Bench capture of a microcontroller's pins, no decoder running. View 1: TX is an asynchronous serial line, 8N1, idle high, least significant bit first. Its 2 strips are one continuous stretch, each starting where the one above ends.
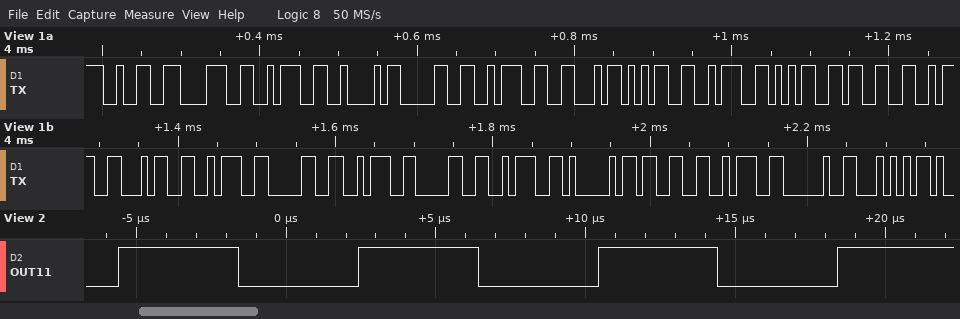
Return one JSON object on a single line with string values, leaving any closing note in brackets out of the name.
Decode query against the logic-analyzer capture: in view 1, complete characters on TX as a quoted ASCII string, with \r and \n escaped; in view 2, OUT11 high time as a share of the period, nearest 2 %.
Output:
{"in view 1, complete characters on TX as a quoted ASCII string, with \\r and \\n escaped": "\"28:B0:F5:53:4:0:0:A3: T\"", "in view 2, OUT11 high time as a share of the period, nearest 2 %": "50 %"}
